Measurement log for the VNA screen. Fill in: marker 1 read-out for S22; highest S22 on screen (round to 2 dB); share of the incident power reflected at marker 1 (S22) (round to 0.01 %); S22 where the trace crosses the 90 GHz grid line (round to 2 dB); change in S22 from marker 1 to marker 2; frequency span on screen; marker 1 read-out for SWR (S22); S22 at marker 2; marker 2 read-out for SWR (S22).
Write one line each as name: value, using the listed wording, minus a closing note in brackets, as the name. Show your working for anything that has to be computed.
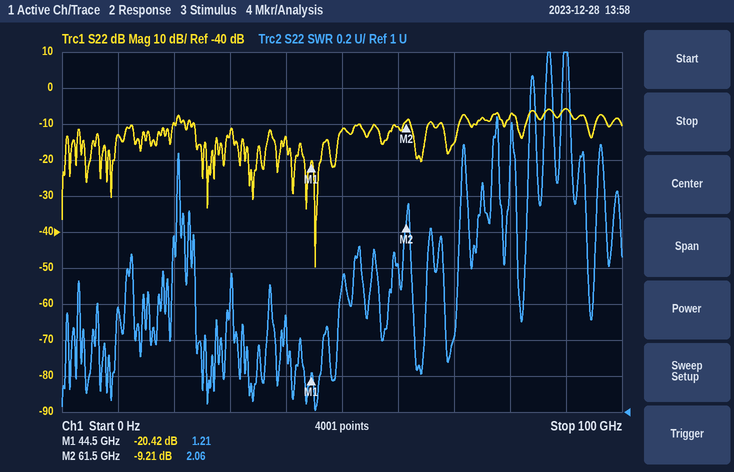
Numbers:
marker 1 read-out for S22: -20.42 dB
highest S22 on screen: -6 dB
share of the incident power reflected at marker 1 (S22): 10^(-20.42/10) ≈ 0.91 %
S22 where the trace crosses the 90 GHz grid line: -6 dB
change in S22 from marker 1 to marker 2: -9.21 − (-20.42) = 11.21 dB
frequency span on screen: 100 GHz
marker 1 read-out for SWR: 1.21
S22 at marker 2: -9.21 dB
marker 2 read-out for SWR: 2.06
